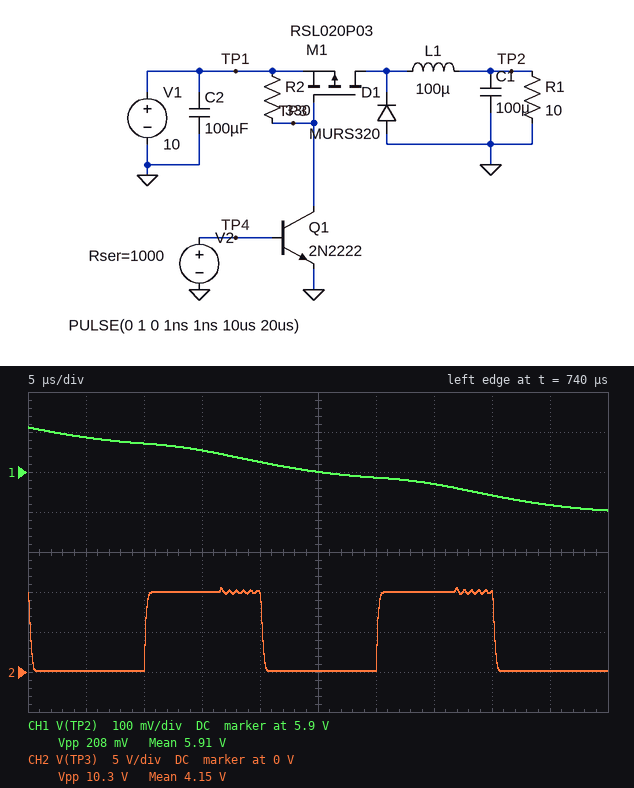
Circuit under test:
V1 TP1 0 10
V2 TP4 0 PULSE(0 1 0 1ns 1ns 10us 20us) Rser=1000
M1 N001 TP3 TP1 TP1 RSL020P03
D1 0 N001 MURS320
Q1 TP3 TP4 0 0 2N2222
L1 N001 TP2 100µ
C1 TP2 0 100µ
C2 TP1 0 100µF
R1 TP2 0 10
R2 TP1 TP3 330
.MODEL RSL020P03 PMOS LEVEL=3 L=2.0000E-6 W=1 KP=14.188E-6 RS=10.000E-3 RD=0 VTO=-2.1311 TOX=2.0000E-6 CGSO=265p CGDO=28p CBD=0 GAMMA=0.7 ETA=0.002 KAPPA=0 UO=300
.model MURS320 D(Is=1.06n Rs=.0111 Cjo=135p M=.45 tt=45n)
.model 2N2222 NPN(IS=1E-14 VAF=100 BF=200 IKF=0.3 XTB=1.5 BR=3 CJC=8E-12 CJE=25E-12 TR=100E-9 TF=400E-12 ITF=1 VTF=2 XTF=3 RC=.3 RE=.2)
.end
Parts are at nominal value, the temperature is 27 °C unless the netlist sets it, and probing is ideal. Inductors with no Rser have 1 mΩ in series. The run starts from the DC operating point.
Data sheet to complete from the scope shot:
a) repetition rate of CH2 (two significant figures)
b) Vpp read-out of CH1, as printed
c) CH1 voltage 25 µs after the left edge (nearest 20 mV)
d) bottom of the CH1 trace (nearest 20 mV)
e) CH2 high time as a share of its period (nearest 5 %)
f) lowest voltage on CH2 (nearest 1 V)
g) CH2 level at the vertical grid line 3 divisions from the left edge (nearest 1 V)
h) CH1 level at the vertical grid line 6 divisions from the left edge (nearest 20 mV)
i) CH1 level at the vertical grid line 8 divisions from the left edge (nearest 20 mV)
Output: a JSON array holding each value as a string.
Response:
["50 kHz", "208 mV", "5.90 V", "5.80 V", "50 %", "0 V", "10 V", "5.88 V", "5.84 V"]
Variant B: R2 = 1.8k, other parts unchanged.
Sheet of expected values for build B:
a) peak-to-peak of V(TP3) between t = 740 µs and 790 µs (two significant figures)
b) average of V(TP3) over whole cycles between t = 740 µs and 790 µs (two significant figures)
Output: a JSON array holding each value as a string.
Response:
["11 V", "4.8 V"]
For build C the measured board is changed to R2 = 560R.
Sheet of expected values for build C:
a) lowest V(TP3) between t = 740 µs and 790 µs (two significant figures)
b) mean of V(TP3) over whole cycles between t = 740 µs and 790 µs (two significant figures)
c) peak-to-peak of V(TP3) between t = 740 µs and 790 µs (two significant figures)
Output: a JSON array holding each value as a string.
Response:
["100 mV", "5.0 V", "11 V"]
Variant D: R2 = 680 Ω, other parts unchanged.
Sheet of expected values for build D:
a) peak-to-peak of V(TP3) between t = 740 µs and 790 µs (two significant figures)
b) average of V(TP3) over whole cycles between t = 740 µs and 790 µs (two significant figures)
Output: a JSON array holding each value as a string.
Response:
["11 V", "5.0 V"]
